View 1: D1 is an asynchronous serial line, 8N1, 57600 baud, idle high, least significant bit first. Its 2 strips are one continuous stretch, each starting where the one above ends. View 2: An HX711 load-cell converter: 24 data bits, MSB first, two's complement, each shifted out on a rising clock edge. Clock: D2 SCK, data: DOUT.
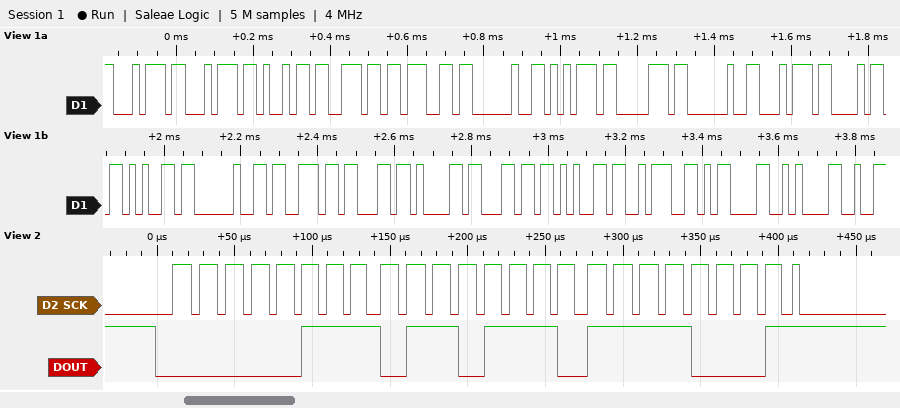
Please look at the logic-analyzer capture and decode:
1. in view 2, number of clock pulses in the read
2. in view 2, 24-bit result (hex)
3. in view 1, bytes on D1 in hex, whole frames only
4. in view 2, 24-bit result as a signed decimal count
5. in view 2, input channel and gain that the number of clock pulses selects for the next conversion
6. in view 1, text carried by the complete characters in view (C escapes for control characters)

25
0x076EF1
74 74 69 6E 67 20 75 70 20 74 68 65 20 73 63 61 6C 65 3A 0D 0A
487153
channel A, gain 128
"tting up the scale:\r\n"
